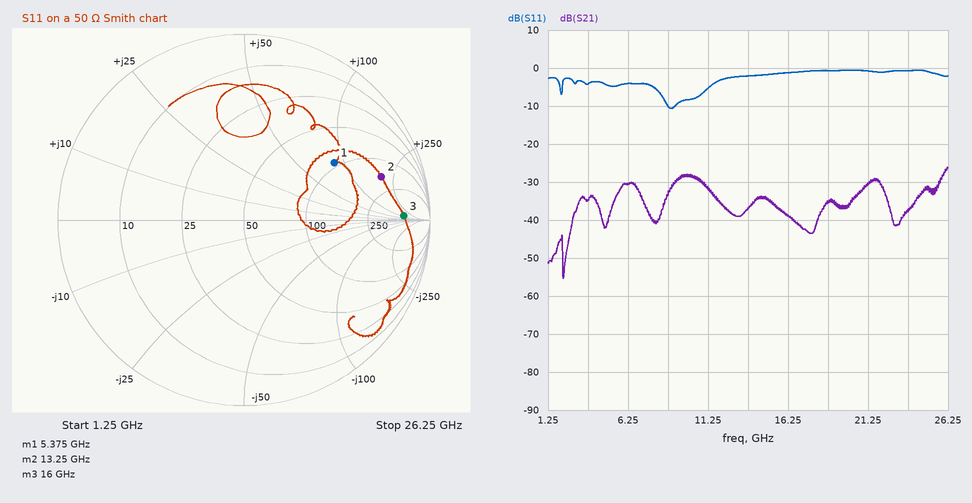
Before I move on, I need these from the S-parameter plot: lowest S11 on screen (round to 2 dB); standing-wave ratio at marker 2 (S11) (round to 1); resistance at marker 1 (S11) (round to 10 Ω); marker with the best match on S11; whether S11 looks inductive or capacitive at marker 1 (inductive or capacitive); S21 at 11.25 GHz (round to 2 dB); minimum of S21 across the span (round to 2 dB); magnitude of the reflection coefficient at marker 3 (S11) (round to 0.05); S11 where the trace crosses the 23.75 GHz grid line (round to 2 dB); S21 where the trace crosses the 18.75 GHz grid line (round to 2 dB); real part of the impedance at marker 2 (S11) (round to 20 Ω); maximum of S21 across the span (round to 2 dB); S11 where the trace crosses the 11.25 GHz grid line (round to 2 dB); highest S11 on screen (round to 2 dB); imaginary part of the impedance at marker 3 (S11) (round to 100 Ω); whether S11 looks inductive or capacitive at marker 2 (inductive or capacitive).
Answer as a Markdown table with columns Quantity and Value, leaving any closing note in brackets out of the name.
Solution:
| Quantity | Value |
|---|---|
| lowest S11 on screen | -10 dB |
| standing-wave ratio at marker 2 (S11) | 8 |
| resistance at marker 1 (S11) | 90 Ω |
| marker with the best match on S11 | marker 1 |
| whether S11 looks inductive or capacitive at marker 1 | inductive |
| S21 at 11.25 GHz | -32 dB |
| minimum of S21 across the span | -56 dB |
| magnitude of the reflection coefficient at marker 3 (S11) | 0.85 |
| S11 where the trace crosses the 23.75 GHz grid line | 0 dB |
| S21 where the trace crosses the 18.75 GHz grid line | -36 dB |
| real part of the impedance at marker 2 (S11) | 160 Ω |
| maximum of S21 across the span | -26 dB |
| S11 where the trace crosses the 11.25 GHz grid line | -6 dB |
| highest S11 on screen | 0 dB |
| imaginary part of the impedance at marker 3 (S11) | +100 Ω |
| whether S11 looks inductive or capacitive at marker 2 | inductive |
